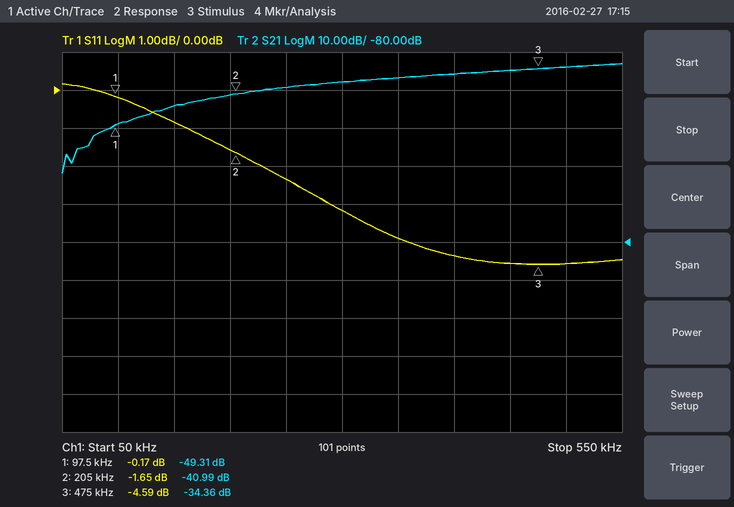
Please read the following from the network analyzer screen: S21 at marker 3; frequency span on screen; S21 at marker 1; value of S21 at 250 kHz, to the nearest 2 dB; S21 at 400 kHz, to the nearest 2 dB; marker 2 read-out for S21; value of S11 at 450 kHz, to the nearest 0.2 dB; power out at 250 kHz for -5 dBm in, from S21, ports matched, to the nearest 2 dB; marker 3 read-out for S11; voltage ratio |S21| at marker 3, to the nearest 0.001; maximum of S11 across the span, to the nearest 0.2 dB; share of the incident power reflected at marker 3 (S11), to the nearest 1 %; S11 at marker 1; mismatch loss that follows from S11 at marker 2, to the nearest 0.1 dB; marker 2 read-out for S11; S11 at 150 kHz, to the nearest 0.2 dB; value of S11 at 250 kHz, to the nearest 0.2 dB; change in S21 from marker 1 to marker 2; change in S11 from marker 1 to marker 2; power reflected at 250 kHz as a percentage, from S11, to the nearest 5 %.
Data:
-34.36 dB
500 kHz
-49.31 dB
-40 dB
-36 dB
-40.99 dB
-4.6 dB
-44 dBm
-4.59 dB
0.019
0.2 dB
35 %
-0.17 dB
5.0 dB
-1.65 dB
-0.8 dB
-2.4 dB
8.32 dB
-1.48 dB
60 %
